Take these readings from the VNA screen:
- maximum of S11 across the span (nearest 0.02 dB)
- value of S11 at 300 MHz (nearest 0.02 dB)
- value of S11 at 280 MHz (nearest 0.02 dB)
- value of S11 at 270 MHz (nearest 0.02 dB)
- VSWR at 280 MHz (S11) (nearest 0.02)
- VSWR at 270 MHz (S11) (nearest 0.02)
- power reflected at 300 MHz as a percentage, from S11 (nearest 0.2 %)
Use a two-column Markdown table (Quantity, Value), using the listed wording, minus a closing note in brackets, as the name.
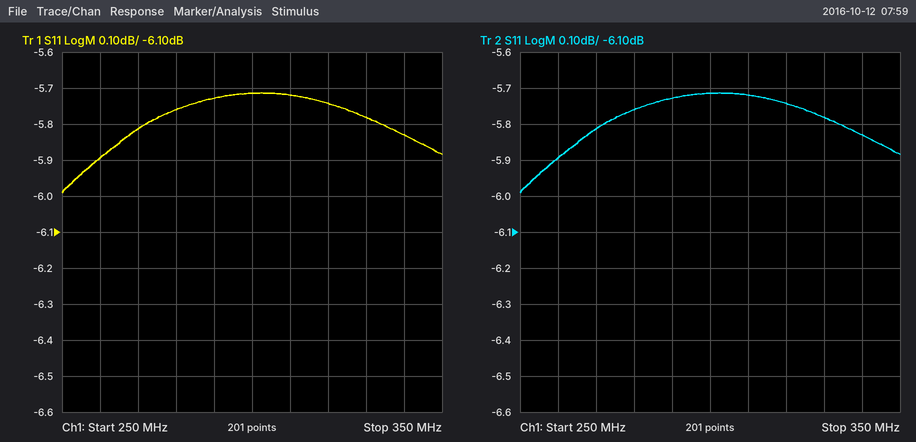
| Quantity | Value |
|---|---|
| maximum of S11 across the span | -5.72 dB |
| value of S11 at 300 MHz | -5.72 dB |
| value of S11 at 280 MHz | -5.76 dB |
| value of S11 at 270 MHz | -5.82 dB |
| VSWR at 280 MHz (S11) | 3.12 |
| VSWR at 270 MHz (S11) | 3.10 |
| power reflected at 300 MHz as a percentage, from S11 | 26.8 % |
